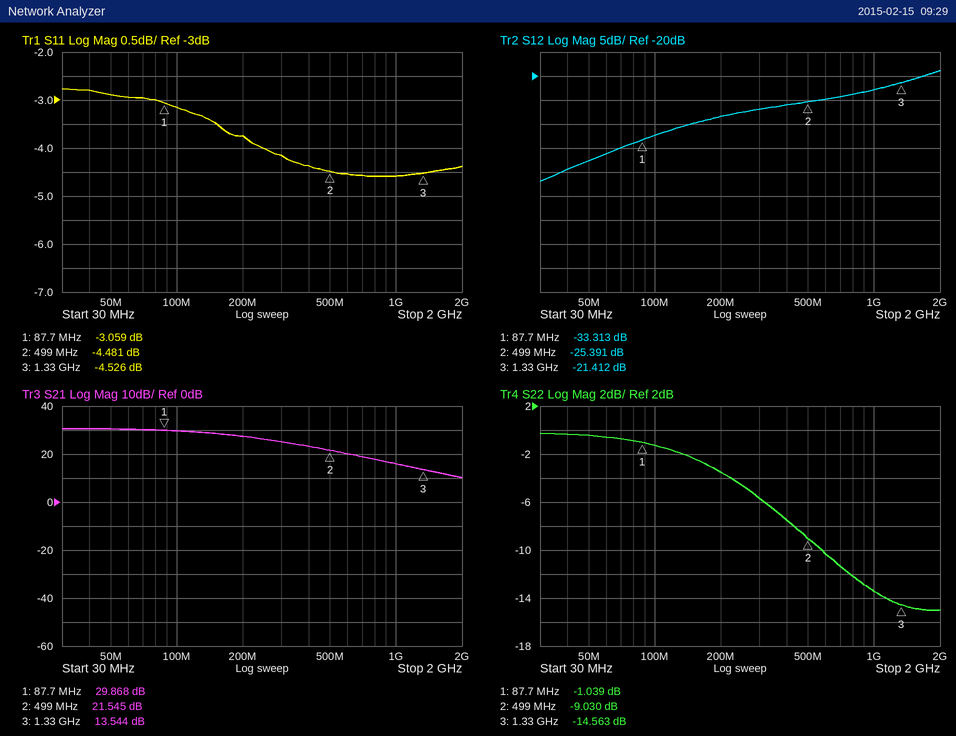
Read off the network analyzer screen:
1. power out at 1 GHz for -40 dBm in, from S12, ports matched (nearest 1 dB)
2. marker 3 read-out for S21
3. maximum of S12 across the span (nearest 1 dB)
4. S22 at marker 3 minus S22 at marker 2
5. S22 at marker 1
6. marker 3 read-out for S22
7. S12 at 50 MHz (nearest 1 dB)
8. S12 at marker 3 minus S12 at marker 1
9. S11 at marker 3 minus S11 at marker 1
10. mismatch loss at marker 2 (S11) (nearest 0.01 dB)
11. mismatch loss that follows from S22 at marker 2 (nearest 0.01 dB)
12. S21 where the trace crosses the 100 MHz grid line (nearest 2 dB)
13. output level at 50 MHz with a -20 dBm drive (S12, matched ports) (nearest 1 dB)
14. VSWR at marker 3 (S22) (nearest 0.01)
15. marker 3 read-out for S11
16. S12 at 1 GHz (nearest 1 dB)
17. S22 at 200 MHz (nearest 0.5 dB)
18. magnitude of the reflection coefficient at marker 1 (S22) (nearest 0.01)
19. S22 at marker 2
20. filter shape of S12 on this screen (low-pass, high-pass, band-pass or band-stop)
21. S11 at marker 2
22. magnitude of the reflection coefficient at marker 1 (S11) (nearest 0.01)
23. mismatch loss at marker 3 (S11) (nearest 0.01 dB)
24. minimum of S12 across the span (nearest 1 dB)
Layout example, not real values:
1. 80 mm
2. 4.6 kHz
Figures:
1. -63 dBm
2. 13.544 dB
3. -19 dB
4. -5.533 dB
5. -1.039 dB
6. -14.563 dB
7. -38 dB
8. 11.901 dB
9. -1.467 dB
10. 1.91 dB
11. 0.58 dB
12. 30 dB
13. -58 dBm
14. 1.46
15. -4.526 dB
16. -23 dB
17. -3.5 dB
18. 0.89
19. -9.030 dB
20. high-pass
21. -4.481 dB
22. 0.70
23. 1.89 dB
24. -42 dB
